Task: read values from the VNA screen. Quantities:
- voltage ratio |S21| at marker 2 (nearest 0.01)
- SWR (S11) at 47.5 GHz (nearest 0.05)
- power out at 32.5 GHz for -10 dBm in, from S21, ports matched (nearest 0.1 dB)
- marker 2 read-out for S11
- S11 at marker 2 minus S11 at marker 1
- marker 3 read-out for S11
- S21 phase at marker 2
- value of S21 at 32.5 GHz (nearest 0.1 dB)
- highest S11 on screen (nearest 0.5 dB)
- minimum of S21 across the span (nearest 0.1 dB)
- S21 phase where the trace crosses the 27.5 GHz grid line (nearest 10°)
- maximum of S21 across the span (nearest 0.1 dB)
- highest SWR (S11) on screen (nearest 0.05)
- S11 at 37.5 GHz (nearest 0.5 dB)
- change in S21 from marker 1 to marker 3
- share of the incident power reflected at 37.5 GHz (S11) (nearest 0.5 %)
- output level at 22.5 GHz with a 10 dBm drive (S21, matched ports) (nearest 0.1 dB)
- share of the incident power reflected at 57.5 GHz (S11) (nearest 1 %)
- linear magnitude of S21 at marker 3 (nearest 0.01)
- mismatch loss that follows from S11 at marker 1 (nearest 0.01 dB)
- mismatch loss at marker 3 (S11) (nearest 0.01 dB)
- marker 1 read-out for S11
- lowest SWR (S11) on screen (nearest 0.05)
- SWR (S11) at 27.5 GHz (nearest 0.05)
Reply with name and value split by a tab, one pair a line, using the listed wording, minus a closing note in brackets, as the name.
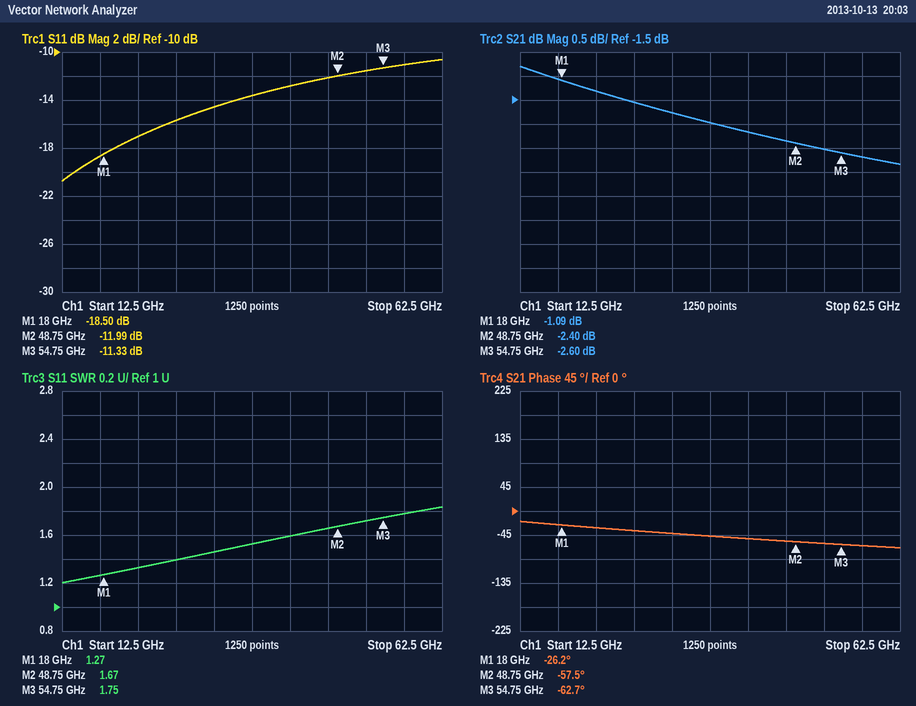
voltage ratio |S21| at marker 2	0.76
SWR (S11) at 47.5 GHz	1.65
power out at 32.5 GHz for -10 dBm in, from S21, ports matched	-11.8 dBm
marker 2 read-out for S11	-11.99 dB
S11 at marker 2 minus S11 at marker 1	6.51 dB
marker 3 read-out for S11	-11.33 dB
S21 phase at marker 2	-57.5°
value of S21 at 32.5 GHz	-1.8 dB
highest S11 on screen	-10.5 dB
minimum of S21 across the span	-2.8 dB
S21 phase where the trace crosses the 27.5 GHz grid line	-40°
maximum of S21 across the span	-0.8 dB
highest SWR (S11) on screen	1.85
S11 at 37.5 GHz	-13.5 dB
change in S21 from marker 1 to marker 3	-1.51 dB
share of the incident power reflected at 37.5 GHz (S11)	4.5 %
output level at 22.5 GHz with a 10 dBm drive (S21, matched ports)	8.7 dBm
share of the incident power reflected at 57.5 GHz (S11)	8 %
linear magnitude of S21 at marker 3	0.74
mismatch loss that follows from S11 at marker 1	0.06 dB
mismatch loss at marker 3 (S11)	0.33 dB
marker 1 read-out for S11	-18.50 dB
lowest SWR (S11) on screen	1.20
SWR (S11) at 27.5 GHz	1.40
